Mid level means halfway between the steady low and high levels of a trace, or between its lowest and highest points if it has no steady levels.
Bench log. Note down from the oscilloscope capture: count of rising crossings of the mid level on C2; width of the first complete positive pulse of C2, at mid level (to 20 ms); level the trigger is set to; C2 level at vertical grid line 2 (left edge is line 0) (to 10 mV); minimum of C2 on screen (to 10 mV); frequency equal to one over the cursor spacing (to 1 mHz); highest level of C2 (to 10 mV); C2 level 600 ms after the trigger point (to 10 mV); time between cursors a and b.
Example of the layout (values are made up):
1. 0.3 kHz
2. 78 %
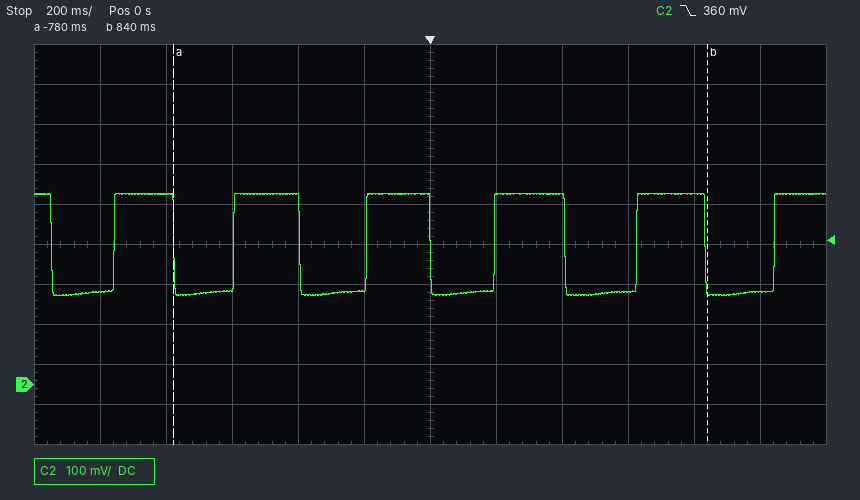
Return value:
1. 6
2. 180 ms
3. 360 mV
4. 480 mV
5. 220 mV
6. 617 mHz
7. 480 mV
8. 230 mV
9. 1.62 s
